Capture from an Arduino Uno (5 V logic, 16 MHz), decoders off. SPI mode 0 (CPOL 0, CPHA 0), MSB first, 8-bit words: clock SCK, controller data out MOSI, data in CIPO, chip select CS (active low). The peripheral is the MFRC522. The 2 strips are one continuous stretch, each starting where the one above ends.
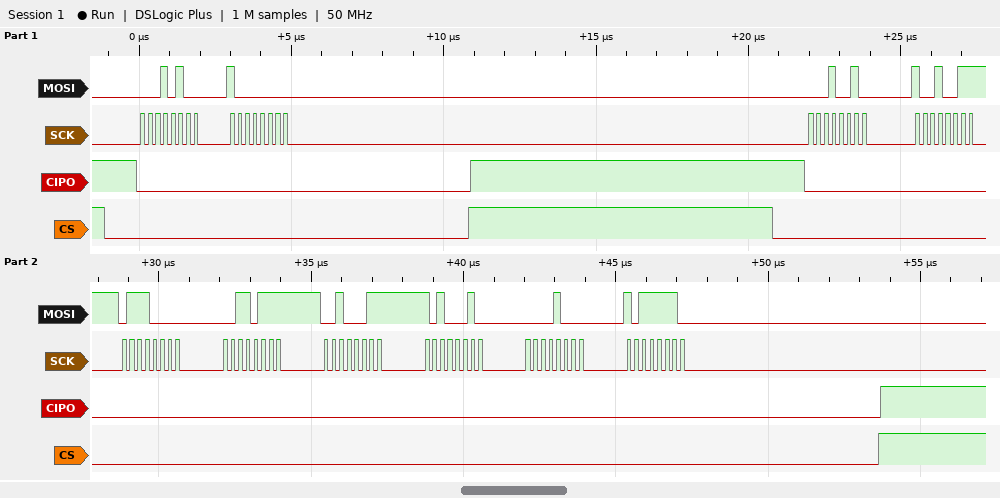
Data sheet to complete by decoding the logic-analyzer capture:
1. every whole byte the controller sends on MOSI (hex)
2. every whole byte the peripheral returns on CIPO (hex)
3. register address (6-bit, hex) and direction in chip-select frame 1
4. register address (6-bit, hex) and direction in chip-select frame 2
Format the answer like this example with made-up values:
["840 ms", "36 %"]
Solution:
["0x14 0x80 0x12 0x93 0x70 0x37 0x23 0xA2 0x08 0xBE", "0x00 0x00 0x00 0x00 0x00 0x00 0x00 0x00 0x00 0x00", "0x0A write", "0x09 write"]
